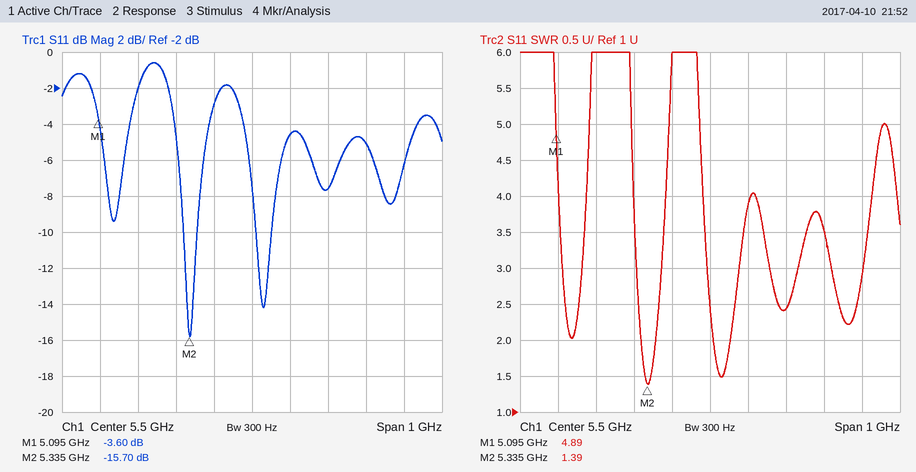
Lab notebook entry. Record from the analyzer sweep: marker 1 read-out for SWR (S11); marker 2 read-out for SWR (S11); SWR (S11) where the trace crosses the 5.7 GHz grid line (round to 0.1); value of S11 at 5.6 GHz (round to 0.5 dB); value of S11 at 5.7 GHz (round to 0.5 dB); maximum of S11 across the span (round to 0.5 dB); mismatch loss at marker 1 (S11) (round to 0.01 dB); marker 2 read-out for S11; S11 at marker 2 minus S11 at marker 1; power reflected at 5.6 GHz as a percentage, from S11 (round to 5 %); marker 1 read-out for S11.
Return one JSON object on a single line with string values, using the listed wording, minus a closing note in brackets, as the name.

{"marker 1 read-out for SWR": "4.89", "marker 2 read-out for SWR": "1.39", "SWR (S11) where the trace crosses the 5.7 GHz grid line": "2.4", "value of S11 at 5.6 GHz": "-4.5 dB", "value of S11 at 5.7 GHz": "-7.5 dB", "maximum of S11 across the span": "-0.5 dB", "mismatch loss at marker 1 (S11)": "2.49 dB", "marker 2 read-out for S11": "-15.70 dB", "S11 at marker 2 minus S11 at marker 1": "-12.10 dB", "power reflected at 5.6 GHz as a percentage, from S11": "35 %", "marker 1 read-out for S11": "-3.60 dB"}
